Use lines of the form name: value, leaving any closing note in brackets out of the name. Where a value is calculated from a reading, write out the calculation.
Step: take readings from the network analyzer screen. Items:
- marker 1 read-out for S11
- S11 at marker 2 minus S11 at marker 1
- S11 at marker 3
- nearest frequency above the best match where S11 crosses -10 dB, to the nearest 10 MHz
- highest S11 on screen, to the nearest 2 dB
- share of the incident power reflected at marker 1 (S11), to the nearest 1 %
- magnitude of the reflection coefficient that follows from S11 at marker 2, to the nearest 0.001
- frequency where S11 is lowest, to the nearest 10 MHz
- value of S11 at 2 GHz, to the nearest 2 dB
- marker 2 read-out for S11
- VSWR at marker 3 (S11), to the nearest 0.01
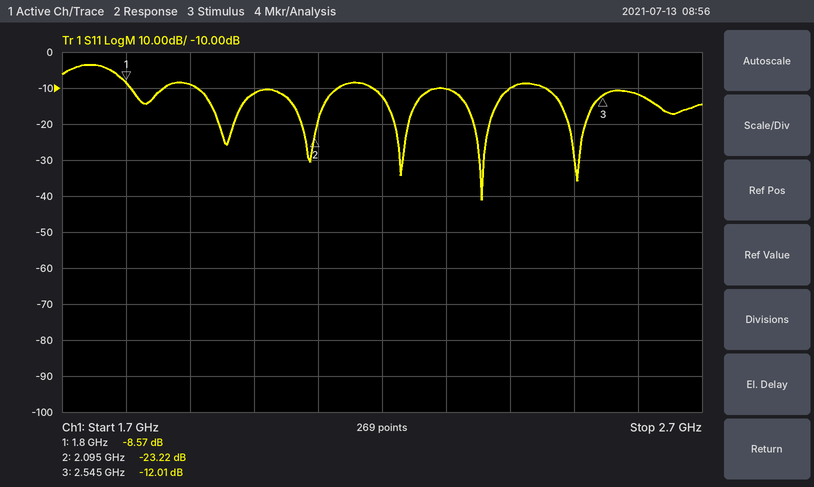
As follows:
marker 1 read-out for S11: -8.57 dB
S11 at marker 2 minus S11 at marker 1: -23.22 − (-8.57) = -14.65 dB
S11 at marker 3: -12.01 dB
nearest frequency above the best match where S11 crosses -10 dB, to the nearest 10 MHz: 2.40 GHz
highest S11 on screen, to the nearest 2 dB: -4 dB
share of the incident power reflected at marker 1 (S11), to the nearest 1 %: 10^(-8.57/10) ≈ 14 %
magnitude of the reflection coefficient that follows from S11 at marker 2, to the nearest 0.001: 10^(-23.22/20) ≈ 0.069
frequency where S11 is lowest, to the nearest 10 MHz: 2.36 GHz
value of S11 at 2 GHz, to the nearest 2 dB: -12 dB
marker 2 read-out for S11: -23.22 dB
VSWR at marker 3 (S11), to the nearest 0.01: (1 + 0.2509)/(1 − 0.2509) ≈ 1.67
